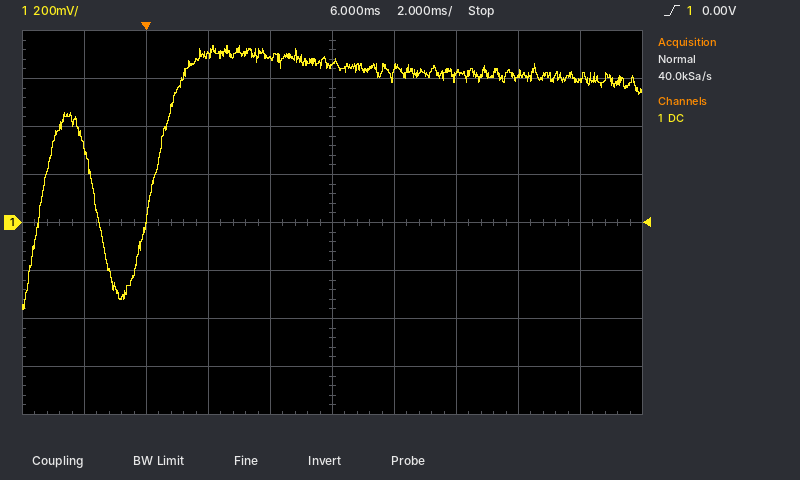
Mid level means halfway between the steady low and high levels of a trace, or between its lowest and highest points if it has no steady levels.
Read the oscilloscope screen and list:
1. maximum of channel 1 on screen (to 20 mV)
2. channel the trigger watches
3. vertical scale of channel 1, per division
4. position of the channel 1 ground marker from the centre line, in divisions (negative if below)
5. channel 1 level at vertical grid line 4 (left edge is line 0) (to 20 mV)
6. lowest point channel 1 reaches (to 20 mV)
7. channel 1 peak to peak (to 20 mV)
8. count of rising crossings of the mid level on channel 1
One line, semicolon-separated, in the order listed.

740 mV; channel 1; 200 mV; 0.0 div; 680 mV; -360 mV; 1.10 V; 2
